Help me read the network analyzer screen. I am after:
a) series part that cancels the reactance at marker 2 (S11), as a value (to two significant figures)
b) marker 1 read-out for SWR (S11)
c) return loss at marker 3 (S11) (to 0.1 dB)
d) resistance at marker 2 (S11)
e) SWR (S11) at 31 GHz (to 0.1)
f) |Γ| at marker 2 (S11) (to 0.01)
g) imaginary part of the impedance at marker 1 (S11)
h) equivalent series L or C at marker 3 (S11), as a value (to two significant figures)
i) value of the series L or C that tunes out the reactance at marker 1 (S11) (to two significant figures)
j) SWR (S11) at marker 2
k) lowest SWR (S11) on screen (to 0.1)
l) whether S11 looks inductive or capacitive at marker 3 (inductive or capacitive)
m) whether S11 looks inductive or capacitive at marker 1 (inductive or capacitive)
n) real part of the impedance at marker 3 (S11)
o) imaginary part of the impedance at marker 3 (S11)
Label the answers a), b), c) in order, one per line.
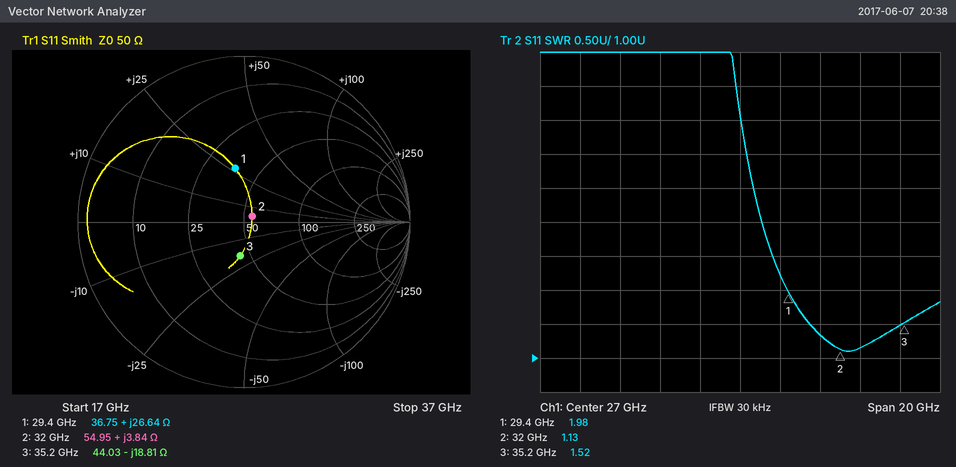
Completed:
a) 1.3 pF
b) 1.98
c) 13.7 dB
d) 54.95 Ω
e) 1.3
f) 0.06
g) +26.64 Ω
h) 240 fF
i) 200 fF
j) 1.13
k) 1.1
l) capacitive
m) inductive
n) 44.03 Ω
o) -18.81 Ω
